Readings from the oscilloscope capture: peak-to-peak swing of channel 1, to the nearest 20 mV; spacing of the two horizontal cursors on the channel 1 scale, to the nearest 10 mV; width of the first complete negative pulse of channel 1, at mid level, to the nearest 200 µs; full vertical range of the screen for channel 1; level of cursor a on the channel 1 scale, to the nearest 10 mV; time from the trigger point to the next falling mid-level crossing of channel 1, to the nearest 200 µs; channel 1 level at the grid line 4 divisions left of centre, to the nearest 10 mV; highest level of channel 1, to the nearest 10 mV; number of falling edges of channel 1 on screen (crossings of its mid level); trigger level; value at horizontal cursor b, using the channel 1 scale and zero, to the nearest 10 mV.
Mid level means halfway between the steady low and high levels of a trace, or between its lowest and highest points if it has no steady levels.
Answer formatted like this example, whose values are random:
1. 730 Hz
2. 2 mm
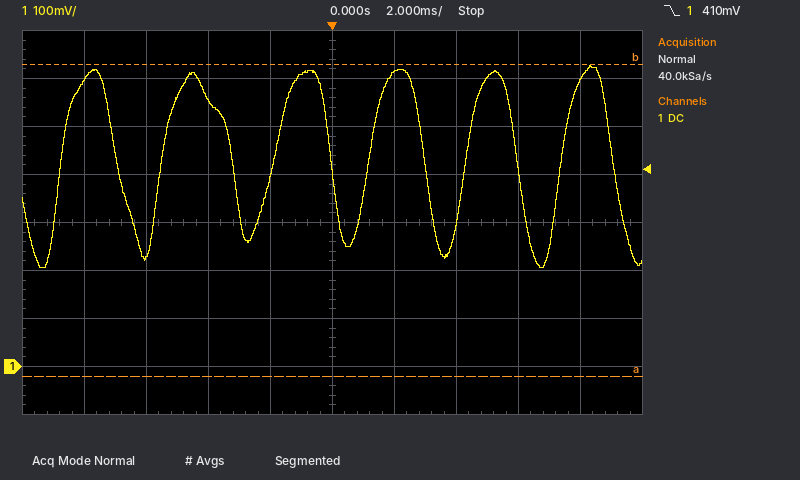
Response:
1. 420 mV
2. 650 mV
3. 1.4 ms
4. 800 mV
5. -20 mV
6. 3.0 ms
7. 600 mV
8. 630 mV
9. 6
10. 410 mV
11. 630 mV
